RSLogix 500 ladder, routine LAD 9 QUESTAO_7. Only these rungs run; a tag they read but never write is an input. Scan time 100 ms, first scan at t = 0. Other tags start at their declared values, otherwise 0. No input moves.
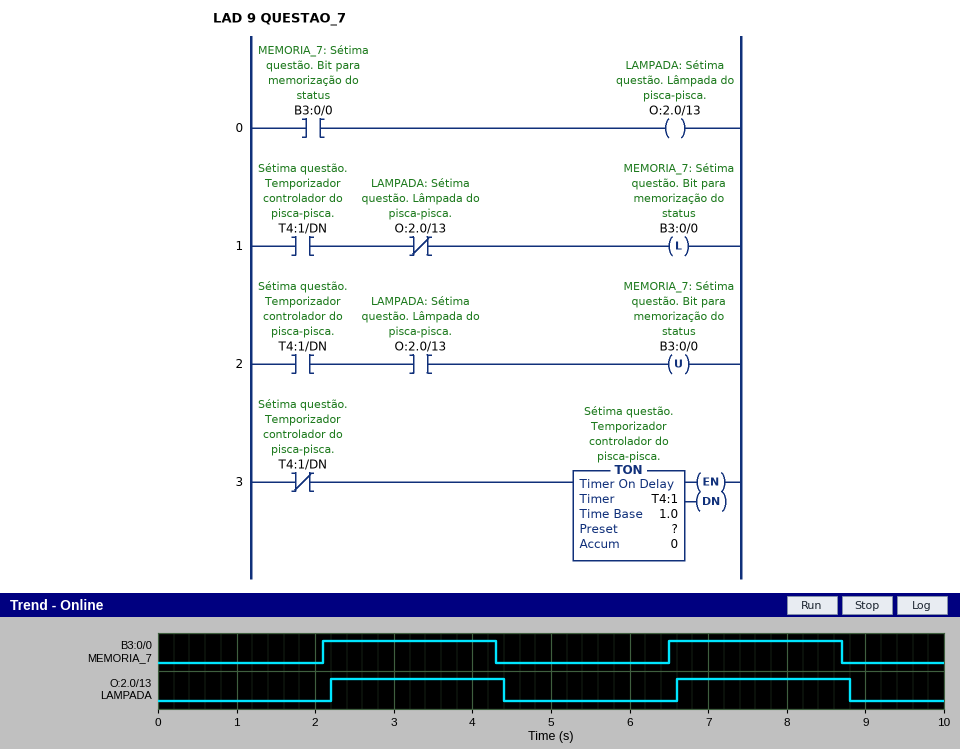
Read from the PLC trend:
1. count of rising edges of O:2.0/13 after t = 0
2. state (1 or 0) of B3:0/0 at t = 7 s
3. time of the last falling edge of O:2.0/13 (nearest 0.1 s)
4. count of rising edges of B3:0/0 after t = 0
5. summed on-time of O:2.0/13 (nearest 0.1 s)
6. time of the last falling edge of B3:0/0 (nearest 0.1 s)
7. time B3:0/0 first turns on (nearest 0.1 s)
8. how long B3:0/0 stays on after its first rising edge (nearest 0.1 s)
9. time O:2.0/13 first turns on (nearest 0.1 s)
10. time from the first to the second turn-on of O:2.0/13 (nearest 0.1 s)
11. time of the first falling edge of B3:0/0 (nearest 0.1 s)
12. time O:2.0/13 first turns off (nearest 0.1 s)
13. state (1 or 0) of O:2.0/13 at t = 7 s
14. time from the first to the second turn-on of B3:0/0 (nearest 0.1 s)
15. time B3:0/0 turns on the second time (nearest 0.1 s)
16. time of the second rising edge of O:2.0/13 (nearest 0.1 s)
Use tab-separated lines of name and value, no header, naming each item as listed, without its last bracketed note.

count of rising edges of O:2.0/13 after t = 0	2
state (1 or 0) of B3:0/0 at t = 7 s	1
time of the last falling edge of O:2.0/13	8.8 s
count of rising edges of B3:0/0 after t = 0	2
summed on-time of O:2.0/13	4.4 s
time of the last falling edge of B3:0/0	8.7 s
time B3:0/0 first turns on	2.1 s
how long B3:0/0 stays on after its first rising edge	2.2 s
time O:2.0/13 first turns on	2.2 s
time from the first to the second turn-on of O:2.0/13	4.4 s
time of the first falling edge of B3:0/0	4.3 s
time O:2.0/13 first turns off	4.4 s
state (1 or 0) of O:2.0/13 at t = 7 s	1
time from the first to the second turn-on of B3:0/0	4.4 s
time B3:0/0 turns on the second time	6.5 s
time of the second rising edge of O:2.0/13	6.6 s
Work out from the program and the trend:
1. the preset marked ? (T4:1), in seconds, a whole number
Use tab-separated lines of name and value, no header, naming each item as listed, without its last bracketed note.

the preset marked ? (T4:1), in seconds, a whole number	2 s
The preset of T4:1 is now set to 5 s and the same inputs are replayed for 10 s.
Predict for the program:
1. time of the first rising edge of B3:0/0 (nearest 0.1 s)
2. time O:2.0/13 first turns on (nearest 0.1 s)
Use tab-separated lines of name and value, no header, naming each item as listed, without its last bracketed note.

time of the first rising edge of B3:0/0	5.1 s
time O:2.0/13 first turns on	5.2 s
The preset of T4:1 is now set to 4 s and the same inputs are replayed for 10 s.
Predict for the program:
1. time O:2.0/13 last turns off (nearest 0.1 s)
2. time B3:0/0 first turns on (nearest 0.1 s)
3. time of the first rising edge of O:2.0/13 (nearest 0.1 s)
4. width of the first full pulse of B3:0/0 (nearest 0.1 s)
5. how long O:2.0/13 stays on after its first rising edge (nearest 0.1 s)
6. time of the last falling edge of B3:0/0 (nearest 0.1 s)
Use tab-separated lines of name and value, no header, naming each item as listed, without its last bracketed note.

time O:2.0/13 last turns off	8.4 s
time B3:0/0 first turns on	4.1 s
time of the first rising edge of O:2.0/13	4.2 s
width of the first full pulse of B3:0/0	4.2 s
how long O:2.0/13 stays on after its first rising edge	4.2 s
time of the last falling edge of B3:0/0	8.3 s
